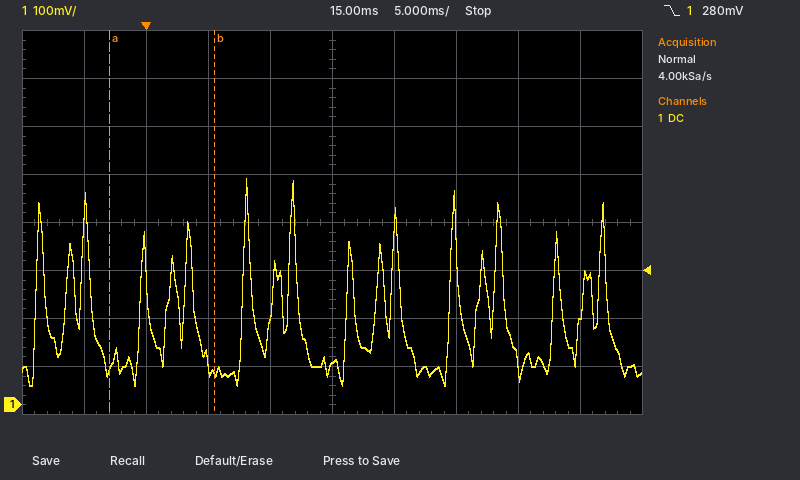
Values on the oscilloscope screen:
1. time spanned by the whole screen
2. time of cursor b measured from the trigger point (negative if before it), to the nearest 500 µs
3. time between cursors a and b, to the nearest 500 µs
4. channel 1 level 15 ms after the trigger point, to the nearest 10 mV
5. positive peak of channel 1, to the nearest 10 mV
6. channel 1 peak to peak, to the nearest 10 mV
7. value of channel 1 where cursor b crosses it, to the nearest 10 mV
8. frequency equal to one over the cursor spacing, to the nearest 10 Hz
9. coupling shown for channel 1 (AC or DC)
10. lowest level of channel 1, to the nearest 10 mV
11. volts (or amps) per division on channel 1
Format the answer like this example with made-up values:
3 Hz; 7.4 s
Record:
50 ms; +5.5 ms; 8.5 ms; 80 mV; 470 mV; 430 mV; 70 mV; 120 Hz; DC; 40 mV; 100 mV
